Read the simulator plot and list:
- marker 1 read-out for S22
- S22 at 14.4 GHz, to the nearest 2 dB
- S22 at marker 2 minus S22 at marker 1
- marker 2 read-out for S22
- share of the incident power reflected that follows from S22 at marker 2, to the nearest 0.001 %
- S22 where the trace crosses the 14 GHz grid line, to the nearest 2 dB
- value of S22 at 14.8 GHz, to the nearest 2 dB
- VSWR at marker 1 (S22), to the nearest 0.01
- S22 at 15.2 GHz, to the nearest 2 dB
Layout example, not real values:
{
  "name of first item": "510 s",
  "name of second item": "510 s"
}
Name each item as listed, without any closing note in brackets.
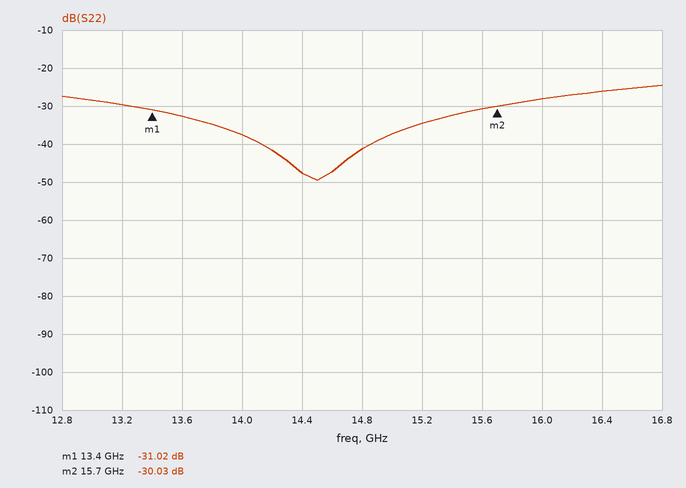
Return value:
{
  "marker 1 read-out for S22": "-31.02 dB",
  "S22 at 14.4 GHz, to the nearest 2 dB": "-48 dB",
  "S22 at marker 2 minus S22 at marker 1": "0.99 dB",
  "marker 2 read-out for S22": "-30.03 dB",
  "share of the incident power reflected that follows from S22 at marker 2, to the nearest 0.001 %": "0.099 %",
  "S22 where the trace crosses the 14 GHz grid line, to the nearest 2 dB": "-38 dB",
  "value of S22 at 14.8 GHz, to the nearest 2 dB": "-42 dB",
  "VSWR at marker 1 (S22), to the nearest 0.01": "1.06",
  "S22 at 15.2 GHz, to the nearest 2 dB": "-34 dB"
}
